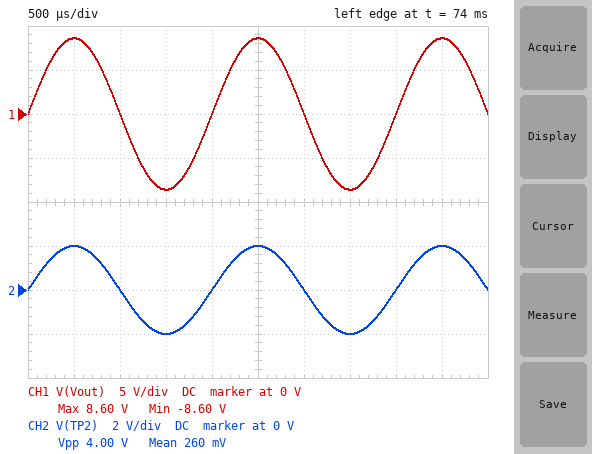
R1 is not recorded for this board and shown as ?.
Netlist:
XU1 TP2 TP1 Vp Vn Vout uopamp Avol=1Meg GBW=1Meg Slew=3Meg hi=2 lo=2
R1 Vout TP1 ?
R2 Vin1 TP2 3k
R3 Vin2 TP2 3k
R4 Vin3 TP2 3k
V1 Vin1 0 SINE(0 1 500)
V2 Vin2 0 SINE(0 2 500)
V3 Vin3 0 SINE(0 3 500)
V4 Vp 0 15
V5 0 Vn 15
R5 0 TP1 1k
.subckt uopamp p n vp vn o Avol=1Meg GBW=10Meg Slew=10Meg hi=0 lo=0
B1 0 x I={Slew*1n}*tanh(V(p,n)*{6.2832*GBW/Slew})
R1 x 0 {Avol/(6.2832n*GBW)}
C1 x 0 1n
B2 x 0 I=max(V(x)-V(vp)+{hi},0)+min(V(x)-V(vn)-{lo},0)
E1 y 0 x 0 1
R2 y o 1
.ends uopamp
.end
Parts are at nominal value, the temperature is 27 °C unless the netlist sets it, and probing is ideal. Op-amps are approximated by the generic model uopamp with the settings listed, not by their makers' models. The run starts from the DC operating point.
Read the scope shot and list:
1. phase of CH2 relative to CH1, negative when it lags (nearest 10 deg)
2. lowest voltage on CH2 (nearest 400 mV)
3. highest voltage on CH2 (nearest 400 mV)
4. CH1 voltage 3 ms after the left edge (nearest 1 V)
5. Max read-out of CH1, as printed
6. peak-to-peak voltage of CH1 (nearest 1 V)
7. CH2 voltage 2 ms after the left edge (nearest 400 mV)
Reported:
0 deg
-2.0 V
2.0 V
0 V
8.60 V
17 V
0 V
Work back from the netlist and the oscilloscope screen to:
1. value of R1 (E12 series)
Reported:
3.3 kΩ
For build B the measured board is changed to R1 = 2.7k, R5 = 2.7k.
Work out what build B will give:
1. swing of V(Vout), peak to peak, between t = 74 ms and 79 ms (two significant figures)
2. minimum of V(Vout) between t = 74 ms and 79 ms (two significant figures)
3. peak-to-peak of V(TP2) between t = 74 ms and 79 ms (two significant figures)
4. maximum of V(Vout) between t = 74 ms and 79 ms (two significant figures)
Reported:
8.0 V
-4.0 V
4.0 V
4.0 V
